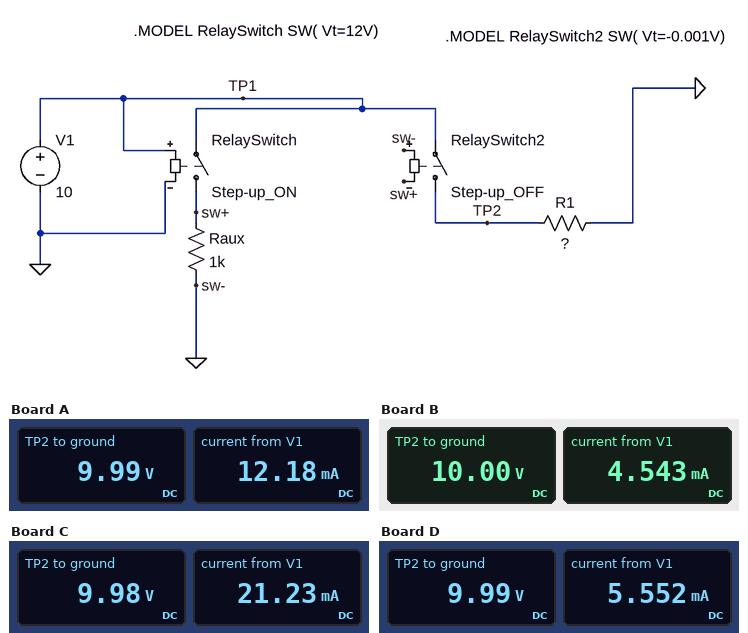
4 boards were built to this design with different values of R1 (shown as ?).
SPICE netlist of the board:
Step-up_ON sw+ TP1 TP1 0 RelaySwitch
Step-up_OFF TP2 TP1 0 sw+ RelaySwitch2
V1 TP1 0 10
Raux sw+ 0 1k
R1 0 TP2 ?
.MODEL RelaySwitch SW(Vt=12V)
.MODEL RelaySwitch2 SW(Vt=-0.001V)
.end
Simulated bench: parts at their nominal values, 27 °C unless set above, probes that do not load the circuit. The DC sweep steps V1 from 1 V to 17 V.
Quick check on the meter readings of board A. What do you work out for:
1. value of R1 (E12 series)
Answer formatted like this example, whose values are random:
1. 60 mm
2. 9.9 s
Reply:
1. 820 Ω
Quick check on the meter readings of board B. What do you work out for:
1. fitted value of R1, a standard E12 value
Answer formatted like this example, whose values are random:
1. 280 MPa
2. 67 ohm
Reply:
1. 2.2 kΩ
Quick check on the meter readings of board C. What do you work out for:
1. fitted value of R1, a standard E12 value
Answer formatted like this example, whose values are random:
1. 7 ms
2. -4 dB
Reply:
1. 470 Ω
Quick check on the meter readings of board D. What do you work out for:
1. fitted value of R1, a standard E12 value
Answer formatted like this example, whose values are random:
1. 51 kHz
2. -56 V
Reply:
1. 1.8 kΩ
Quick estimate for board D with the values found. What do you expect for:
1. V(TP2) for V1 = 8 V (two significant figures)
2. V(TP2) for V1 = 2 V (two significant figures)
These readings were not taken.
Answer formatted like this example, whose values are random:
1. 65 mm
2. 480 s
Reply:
1. 8.0 V
2. 2.0 V
